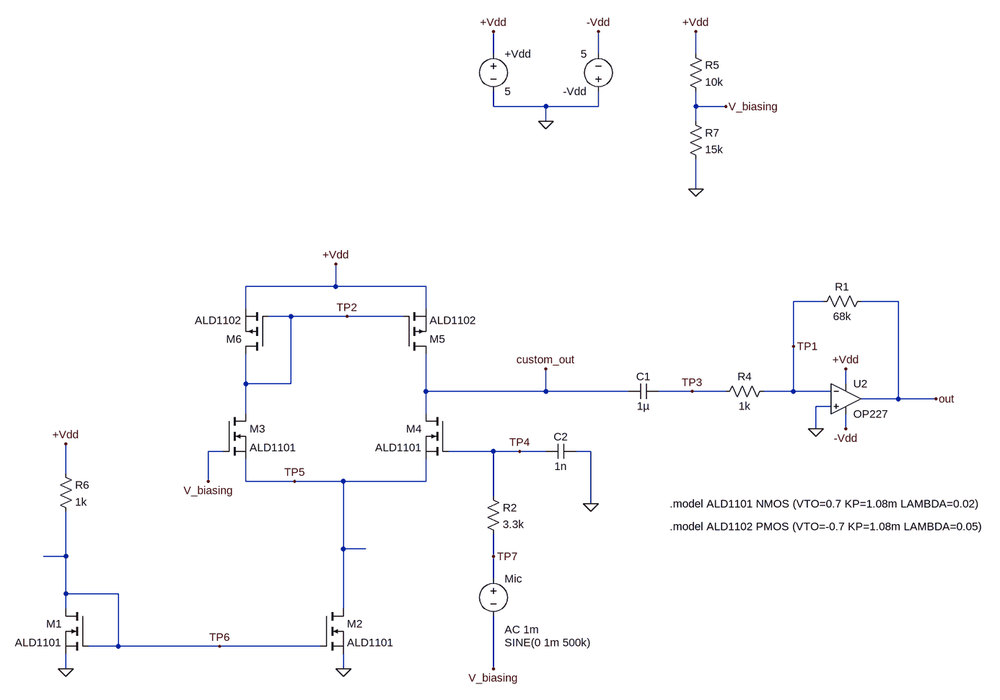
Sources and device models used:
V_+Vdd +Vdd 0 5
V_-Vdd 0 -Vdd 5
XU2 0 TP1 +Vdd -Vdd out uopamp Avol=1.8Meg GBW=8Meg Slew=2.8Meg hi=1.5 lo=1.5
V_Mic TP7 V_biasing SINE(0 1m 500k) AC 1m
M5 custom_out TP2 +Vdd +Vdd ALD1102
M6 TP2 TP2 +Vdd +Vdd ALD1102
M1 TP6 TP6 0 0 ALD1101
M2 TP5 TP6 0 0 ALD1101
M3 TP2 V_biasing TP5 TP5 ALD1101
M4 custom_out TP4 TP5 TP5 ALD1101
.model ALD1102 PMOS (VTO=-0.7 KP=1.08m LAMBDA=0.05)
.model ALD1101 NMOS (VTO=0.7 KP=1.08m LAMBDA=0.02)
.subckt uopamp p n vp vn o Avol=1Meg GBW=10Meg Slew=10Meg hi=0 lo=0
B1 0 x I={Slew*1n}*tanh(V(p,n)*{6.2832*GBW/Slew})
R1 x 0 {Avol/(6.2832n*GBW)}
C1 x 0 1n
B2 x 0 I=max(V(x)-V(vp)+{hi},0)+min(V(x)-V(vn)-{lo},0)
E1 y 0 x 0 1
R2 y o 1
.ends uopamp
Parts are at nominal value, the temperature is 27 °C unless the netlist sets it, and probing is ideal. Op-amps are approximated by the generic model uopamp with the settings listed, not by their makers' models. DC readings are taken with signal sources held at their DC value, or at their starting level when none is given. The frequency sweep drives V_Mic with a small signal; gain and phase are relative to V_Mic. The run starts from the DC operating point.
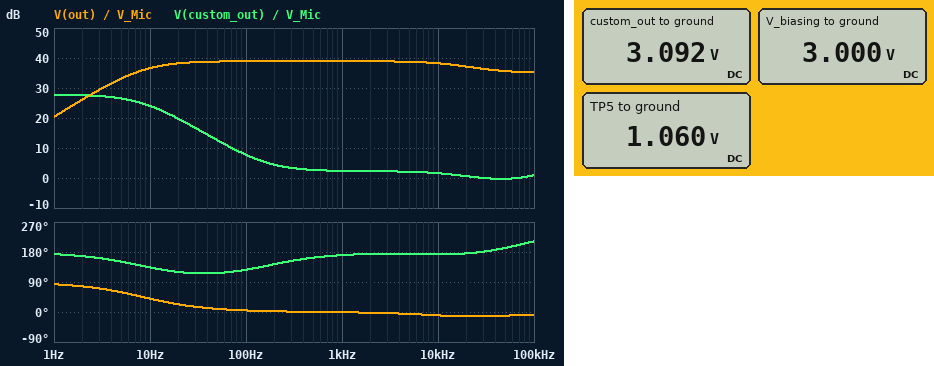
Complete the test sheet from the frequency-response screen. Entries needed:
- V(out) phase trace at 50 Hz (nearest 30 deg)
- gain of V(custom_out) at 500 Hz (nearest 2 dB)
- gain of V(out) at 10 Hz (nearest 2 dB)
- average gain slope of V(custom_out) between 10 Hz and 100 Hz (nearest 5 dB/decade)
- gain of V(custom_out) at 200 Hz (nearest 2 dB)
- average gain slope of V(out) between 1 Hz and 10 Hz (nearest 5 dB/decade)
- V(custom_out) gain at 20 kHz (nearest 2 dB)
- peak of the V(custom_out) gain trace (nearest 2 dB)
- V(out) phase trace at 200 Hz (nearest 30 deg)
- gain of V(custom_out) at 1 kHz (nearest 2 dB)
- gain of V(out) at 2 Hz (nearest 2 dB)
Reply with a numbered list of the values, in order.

1. 0 deg
2. 2 dB
3. 36 dB
4. -15 dB/decade
5. 4 dB
6. 15 dB/decade
7. 0 dB
8. 28 dB
9. 0 deg
10. 2 dB
11. 26 dB
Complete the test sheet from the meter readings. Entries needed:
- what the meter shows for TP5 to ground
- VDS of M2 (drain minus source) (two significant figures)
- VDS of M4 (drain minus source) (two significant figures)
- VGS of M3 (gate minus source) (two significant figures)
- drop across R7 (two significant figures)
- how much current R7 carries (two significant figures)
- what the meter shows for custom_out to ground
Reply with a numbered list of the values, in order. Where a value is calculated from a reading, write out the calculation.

1. 1.060 V
2. 1.06 V = 1.1 V
3. 3.092 V - 1.06 V = 2.0 V
4. 3 V - 1.06 V = 1.9 V
5. 3 V = 3.0 V
6. (3 V) / 15 kΩ = 200 µA
7. 3.092 V
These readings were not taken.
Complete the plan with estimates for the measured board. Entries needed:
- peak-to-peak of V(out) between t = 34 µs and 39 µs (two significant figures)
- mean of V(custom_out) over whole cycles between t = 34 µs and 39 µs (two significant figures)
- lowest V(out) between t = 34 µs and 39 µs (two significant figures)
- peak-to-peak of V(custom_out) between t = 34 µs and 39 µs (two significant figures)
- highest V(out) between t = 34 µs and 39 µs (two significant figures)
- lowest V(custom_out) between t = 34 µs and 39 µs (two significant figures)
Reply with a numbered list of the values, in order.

1. 110 mV
2. 3.1 V
3. -54 mV
4. 7.1 mV
5. 54 mV
6. 3.1 V
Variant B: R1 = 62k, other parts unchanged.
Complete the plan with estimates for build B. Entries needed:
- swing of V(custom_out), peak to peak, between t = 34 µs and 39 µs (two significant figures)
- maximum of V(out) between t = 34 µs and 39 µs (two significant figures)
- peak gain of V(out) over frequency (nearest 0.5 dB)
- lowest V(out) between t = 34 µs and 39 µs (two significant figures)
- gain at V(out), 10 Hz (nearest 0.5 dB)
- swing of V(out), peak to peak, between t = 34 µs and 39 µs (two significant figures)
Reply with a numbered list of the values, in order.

1. 6.5 mV
2. 50 mV
3. 38.0 dB
4. -50 mV
5. 36.0 dB
6. 100 mV
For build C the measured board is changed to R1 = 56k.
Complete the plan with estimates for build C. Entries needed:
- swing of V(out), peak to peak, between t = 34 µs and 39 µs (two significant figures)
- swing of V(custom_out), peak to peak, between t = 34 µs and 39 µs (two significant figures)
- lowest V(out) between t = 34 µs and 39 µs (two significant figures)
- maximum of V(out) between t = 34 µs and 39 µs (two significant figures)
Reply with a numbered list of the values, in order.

1. 90 mV
2. 6.0 mV
3. -45 mV
4. 45 mV
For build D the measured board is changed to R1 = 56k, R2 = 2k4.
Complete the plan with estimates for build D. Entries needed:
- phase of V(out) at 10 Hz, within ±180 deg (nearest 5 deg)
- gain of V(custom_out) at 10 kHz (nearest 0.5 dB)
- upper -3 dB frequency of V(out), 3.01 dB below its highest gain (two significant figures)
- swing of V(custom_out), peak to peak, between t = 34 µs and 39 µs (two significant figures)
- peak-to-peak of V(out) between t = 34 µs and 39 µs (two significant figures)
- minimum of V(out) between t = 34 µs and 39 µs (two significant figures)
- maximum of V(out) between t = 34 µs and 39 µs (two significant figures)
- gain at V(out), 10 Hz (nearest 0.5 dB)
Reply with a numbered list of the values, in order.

1. 40 deg
2. 2.0 dB
3. 190 kHz
4. 6.6 mV
5. 100 mV
6. -50 mV
7. 50 mV
8. 35.0 dB
